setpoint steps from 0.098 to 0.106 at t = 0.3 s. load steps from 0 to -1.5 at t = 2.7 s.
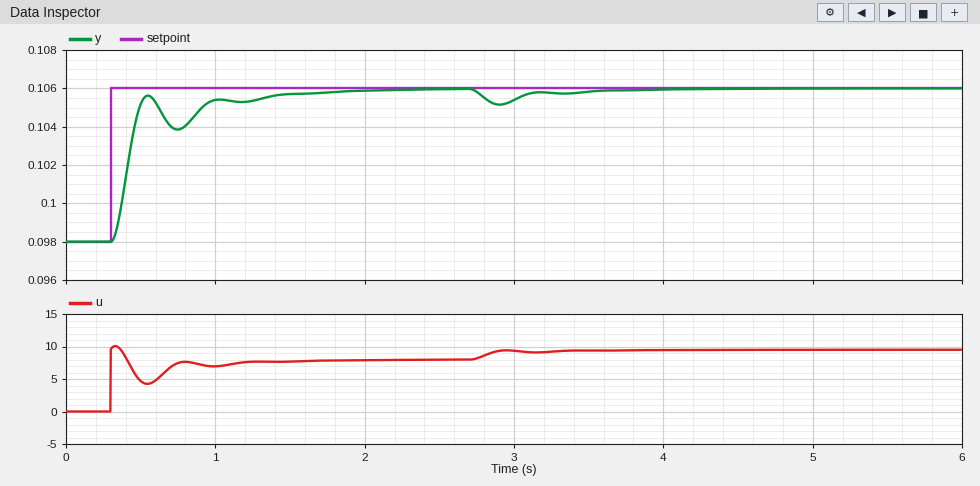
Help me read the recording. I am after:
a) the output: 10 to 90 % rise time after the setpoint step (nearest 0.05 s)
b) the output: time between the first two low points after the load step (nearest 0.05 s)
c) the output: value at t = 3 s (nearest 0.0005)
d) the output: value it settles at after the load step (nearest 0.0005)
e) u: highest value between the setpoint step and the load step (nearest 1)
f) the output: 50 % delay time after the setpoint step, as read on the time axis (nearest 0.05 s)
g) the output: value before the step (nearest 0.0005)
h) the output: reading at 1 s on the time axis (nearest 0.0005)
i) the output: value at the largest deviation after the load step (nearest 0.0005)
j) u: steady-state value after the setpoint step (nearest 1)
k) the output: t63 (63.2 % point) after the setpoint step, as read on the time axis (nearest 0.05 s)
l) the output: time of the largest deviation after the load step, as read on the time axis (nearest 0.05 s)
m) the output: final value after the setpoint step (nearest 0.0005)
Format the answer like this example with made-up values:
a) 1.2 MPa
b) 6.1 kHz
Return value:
a) 0.15 s
b) 0.45 s
c) 0.1055
d) 0.1060
e) 10
f) 0.40 s
g) 0.0980
h) 0.1055
i) 0.1050
j) 8
k) 0.45 s
l) 2.90 s
m) 0.1060
